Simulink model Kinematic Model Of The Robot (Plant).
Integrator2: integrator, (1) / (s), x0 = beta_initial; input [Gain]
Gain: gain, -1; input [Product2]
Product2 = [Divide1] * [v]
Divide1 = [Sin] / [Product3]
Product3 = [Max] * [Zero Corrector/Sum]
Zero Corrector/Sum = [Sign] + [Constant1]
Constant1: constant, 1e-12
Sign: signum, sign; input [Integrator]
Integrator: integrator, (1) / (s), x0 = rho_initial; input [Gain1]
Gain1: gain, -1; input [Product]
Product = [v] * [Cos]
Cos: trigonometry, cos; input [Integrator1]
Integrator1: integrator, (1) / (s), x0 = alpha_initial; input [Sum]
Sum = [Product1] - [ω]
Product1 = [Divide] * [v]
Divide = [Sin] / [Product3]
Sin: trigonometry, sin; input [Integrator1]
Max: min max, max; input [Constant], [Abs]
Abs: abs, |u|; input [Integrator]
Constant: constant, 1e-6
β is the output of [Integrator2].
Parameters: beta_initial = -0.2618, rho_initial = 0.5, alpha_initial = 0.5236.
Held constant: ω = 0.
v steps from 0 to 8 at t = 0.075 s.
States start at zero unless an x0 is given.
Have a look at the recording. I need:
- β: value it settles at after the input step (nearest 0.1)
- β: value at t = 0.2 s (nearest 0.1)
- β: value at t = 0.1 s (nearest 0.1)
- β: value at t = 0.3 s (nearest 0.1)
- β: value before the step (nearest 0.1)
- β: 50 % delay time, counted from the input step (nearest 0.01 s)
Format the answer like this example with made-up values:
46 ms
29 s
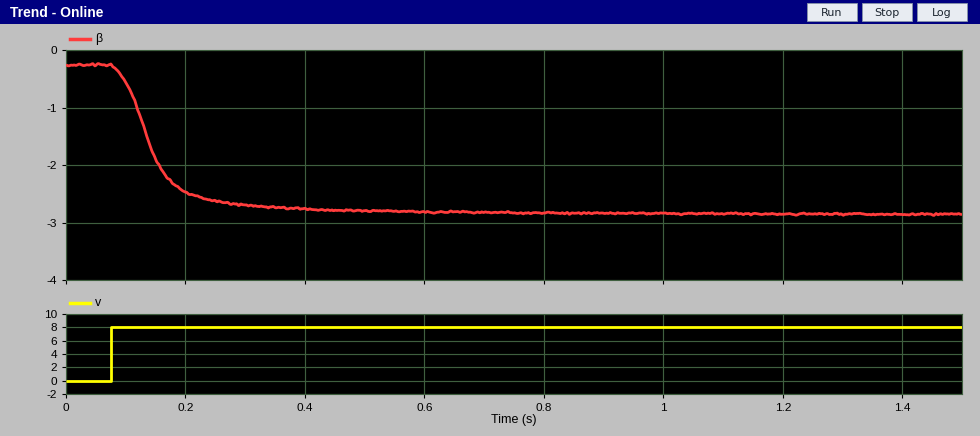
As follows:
-2.9
-2.5
-0.6
-2.7
-0.3
0.06 s
